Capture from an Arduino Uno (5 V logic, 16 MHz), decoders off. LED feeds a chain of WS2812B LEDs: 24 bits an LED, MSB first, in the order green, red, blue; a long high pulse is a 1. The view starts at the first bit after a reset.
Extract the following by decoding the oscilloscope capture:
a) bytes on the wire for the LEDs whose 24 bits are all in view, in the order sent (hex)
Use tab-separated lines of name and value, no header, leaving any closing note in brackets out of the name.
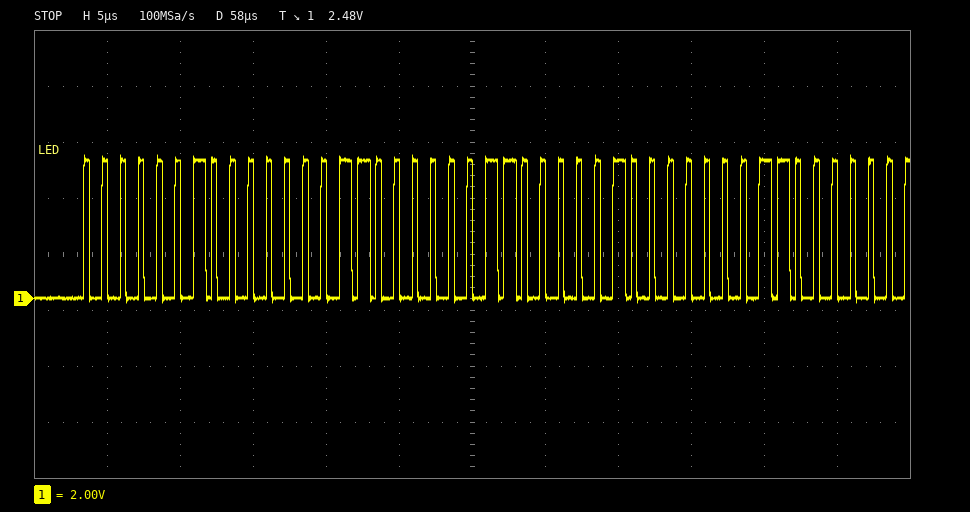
bytes on the wire for the LEDs whose 24 bits are all in view, in the order sent	02 03 03
